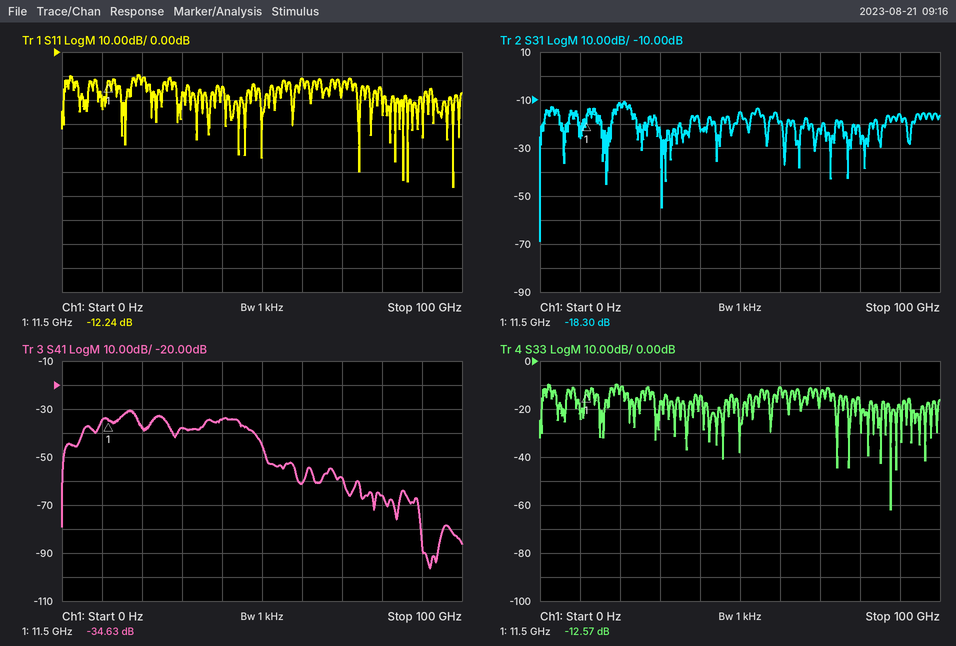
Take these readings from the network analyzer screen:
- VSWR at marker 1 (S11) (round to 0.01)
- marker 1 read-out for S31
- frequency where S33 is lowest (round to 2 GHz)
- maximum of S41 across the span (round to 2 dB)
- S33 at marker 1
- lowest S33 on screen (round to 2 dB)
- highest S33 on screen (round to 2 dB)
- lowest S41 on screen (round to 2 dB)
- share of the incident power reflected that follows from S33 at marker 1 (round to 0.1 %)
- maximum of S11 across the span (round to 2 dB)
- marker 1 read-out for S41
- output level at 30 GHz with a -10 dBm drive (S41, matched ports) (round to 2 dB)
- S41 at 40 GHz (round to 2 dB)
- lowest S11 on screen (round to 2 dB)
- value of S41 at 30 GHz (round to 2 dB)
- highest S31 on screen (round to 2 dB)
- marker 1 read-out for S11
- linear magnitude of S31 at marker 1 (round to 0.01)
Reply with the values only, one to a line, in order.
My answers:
1.65
-18.30 dB
88 GHz
-30 dB
-12.57 dB
-62 dB
-10 dB
-96 dB
5.5 %
-10 dB
-34.63 dB
-48 dBm
-34 dB
-56 dB
-38 dB
-10 dB
-12.24 dB
0.12
